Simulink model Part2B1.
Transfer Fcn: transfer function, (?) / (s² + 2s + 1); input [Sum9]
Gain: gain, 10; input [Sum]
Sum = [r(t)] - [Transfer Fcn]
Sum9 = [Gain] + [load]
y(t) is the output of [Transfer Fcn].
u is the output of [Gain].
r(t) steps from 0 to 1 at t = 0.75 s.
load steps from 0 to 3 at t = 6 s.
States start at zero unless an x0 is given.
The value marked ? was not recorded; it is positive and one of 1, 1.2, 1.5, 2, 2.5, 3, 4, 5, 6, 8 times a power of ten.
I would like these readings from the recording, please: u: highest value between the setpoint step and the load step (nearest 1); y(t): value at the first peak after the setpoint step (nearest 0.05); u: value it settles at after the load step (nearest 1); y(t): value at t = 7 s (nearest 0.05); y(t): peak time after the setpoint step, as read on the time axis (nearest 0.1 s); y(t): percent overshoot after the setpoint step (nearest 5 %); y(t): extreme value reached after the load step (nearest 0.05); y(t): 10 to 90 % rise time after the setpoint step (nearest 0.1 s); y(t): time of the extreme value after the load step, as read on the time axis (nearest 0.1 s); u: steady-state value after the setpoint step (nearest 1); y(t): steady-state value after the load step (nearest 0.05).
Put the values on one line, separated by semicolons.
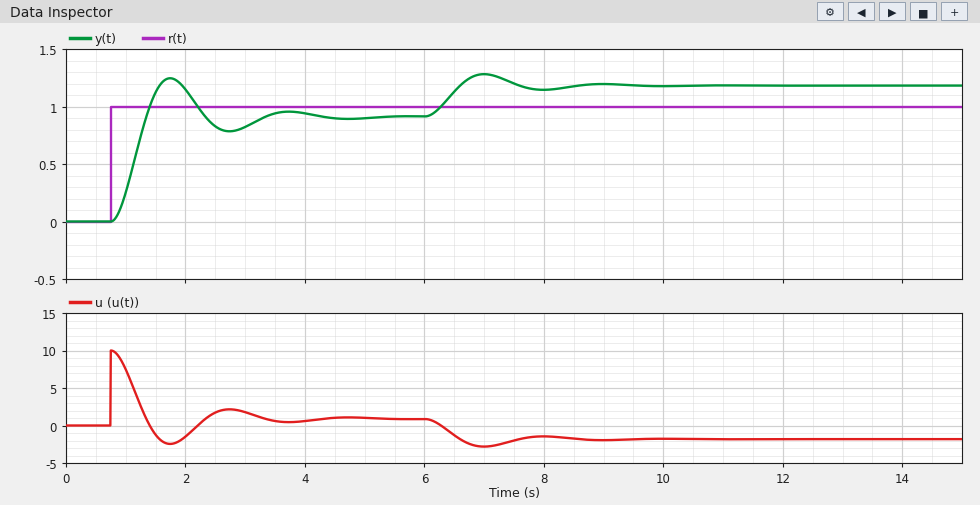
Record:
10; 1.25; -2; 1.30; 1.7 s; 35 %; 1.30; 0.4 s; 7.0 s; 1; 1.20
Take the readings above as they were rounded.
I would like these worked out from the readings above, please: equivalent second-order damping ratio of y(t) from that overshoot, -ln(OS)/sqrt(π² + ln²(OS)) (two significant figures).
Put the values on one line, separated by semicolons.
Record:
0.32
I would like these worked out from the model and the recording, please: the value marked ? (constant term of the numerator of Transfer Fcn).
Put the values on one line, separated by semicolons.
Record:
1
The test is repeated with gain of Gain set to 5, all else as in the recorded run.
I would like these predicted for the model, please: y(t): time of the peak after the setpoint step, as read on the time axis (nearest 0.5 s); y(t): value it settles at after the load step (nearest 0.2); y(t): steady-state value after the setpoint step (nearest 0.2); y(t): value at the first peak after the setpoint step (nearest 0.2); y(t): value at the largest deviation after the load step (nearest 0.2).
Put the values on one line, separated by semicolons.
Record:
2.0 s; 1.4; 0.8; 1.0; 1.4
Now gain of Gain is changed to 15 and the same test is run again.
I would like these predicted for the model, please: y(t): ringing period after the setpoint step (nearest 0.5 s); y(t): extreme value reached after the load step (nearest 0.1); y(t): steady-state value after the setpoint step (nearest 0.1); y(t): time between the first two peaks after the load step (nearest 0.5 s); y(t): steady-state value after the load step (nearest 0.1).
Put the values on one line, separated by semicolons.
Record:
1.5 s; 1.2; 0.9; 1.5 s; 1.1
